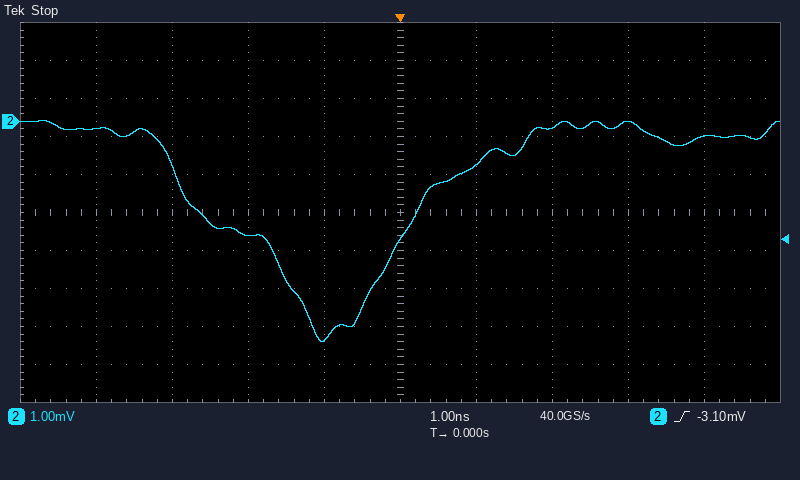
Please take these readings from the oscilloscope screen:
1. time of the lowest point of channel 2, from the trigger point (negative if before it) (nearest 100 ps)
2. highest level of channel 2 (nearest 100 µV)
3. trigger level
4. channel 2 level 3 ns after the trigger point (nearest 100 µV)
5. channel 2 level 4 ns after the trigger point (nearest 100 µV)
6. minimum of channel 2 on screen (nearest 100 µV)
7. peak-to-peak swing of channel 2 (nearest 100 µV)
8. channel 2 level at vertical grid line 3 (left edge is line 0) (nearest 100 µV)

-1.0 ns
0.0 mV
-3.10 mV
0.0 mV
-400 µV
-5.8 mV
5.8 mV
-3.0 mV
